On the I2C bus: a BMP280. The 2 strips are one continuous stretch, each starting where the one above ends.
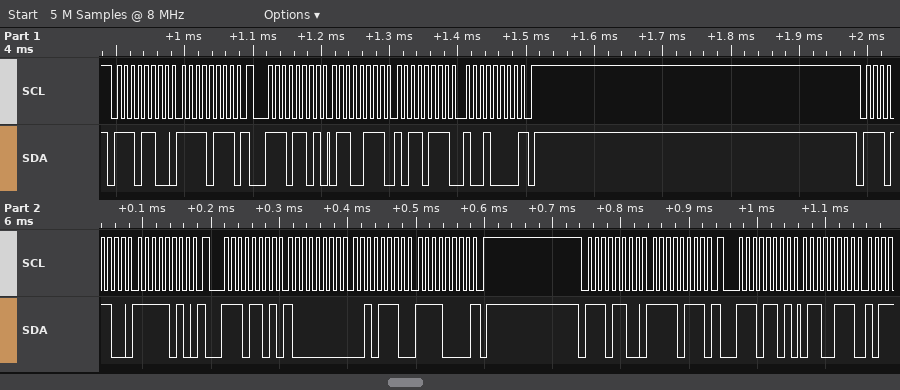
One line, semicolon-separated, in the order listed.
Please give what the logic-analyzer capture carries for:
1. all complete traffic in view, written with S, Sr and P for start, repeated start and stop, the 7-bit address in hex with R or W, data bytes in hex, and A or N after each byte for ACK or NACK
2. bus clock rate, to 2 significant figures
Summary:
S 76W A F7 A Sr 76R A 67 A B7 A 90 N P S 76W A FA A Sr 76R A 80 A 2E A F0 N P S 76W A F7 A Sr 76R A 67 A; 100 kHz
